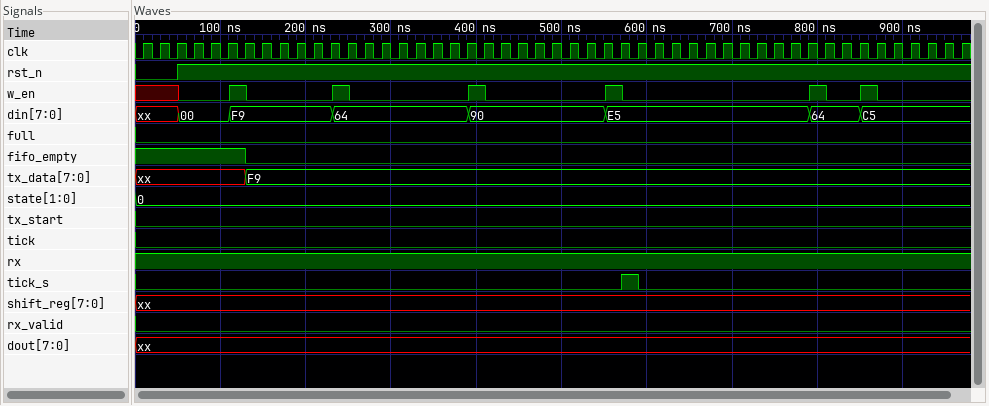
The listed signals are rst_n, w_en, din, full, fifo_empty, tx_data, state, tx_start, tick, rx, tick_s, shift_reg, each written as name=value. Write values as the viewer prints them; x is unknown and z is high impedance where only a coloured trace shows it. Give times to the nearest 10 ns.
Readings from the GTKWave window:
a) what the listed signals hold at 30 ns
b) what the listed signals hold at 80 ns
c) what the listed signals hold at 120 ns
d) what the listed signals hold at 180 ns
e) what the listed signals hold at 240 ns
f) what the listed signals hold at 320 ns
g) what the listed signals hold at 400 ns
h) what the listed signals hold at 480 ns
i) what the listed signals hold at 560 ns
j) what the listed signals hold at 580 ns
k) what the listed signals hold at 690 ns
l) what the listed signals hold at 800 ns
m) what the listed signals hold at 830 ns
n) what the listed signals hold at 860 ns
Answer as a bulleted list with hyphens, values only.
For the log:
- rst_n=0, w_en=x, din=xx, full=0, fifo_empty=1, tx_data=xx, state=0, tx_start=0, tick=0, rx=1, tick_s=0, shift_reg=xx
- rst_n=1, w_en=0, din=00, full=0, fifo_empty=1, tx_data=xx, state=0, tx_start=0, tick=0, rx=1, tick_s=0, shift_reg=xx
- rst_n=1, w_en=1, din=F9, full=0, fifo_empty=1, tx_data=xx, state=0, tx_start=0, tick=0, rx=1, tick_s=0, shift_reg=xx
- rst_n=1, w_en=0, din=F9, full=0, fifo_empty=0, tx_data=F9, state=0, tx_start=0, tick=0, rx=1, tick_s=0, shift_reg=xx
- rst_n=1, w_en=1, din=64, full=0, fifo_empty=0, tx_data=F9, state=0, tx_start=0, tick=0, rx=1, tick_s=0, shift_reg=xx
- rst_n=1, w_en=0, din=64, full=0, fifo_empty=0, tx_data=F9, state=0, tx_start=0, tick=0, rx=1, tick_s=0, shift_reg=xx
- rst_n=1, w_en=1, din=90, full=0, fifo_empty=0, tx_data=F9, state=0, tx_start=0, tick=0, rx=1, tick_s=0, shift_reg=xx
- rst_n=1, w_en=0, din=90, full=0, fifo_empty=0, tx_data=F9, state=0, tx_start=0, tick=0, rx=1, tick_s=0, shift_reg=xx
- rst_n=1, w_en=1, din=E5, full=0, fifo_empty=0, tx_data=F9, state=0, tx_start=0, tick=0, rx=1, tick_s=0, shift_reg=xx
- rst_n=1, w_en=0, din=E5, full=0, fifo_empty=0, tx_data=F9, state=0, tx_start=0, tick=0, rx=1, tick_s=1, shift_reg=xx
- rst_n=1, w_en=0, din=E5, full=0, fifo_empty=0, tx_data=F9, state=0, tx_start=0, tick=0, rx=1, tick_s=0, shift_reg=xx
- rst_n=1, w_en=1, din=64, full=0, fifo_empty=0, tx_data=F9, state=0, tx_start=0, tick=0, rx=1, tick_s=0, shift_reg=xx
- rst_n=1, w_en=0, din=64, full=0, fifo_empty=0, tx_data=F9, state=0, tx_start=0, tick=0, rx=1, tick_s=0, shift_reg=xx
- rst_n=1, w_en=1, din=C5, full=0, fifo_empty=0, tx_data=F9, state=0, tx_start=0, tick=0, rx=1, tick_s=0, shift_reg=xx
